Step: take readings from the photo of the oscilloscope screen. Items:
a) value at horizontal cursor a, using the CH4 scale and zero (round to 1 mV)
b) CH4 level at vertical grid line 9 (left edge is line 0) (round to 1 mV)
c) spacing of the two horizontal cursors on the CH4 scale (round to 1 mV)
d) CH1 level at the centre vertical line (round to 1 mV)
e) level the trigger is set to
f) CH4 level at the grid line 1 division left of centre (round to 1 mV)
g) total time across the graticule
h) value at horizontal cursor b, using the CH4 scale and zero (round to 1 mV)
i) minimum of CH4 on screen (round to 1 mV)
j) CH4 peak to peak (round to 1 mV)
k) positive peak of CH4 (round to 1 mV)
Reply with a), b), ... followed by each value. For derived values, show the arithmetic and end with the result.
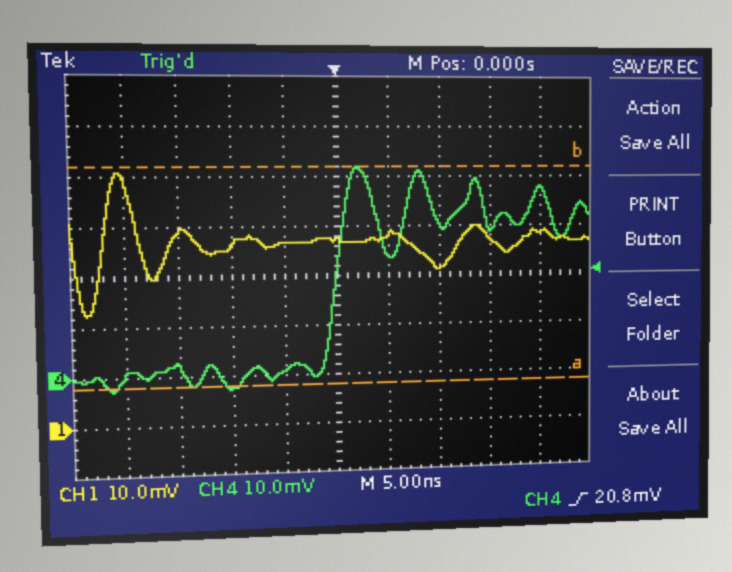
a) -2 mV
b) 37 mV
c) 44 mV
d) 37 mV
e) 20.8 mV
f) 1 mV
g) 50 ns
h) 42 mV
i) -3 mV
j) 42 mV − (-3 mV) = 45 mV
k) 42 mV
